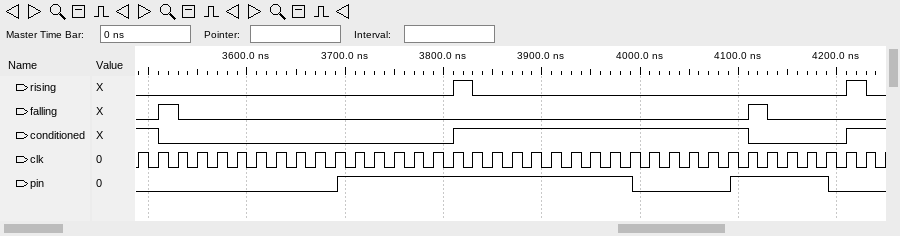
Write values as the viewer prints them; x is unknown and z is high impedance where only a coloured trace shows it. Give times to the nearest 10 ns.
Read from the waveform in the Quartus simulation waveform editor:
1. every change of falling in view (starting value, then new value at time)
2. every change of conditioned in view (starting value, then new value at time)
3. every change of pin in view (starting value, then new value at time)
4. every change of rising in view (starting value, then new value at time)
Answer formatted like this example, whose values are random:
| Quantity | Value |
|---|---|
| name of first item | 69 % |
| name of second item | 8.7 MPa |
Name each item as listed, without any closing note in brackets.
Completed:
| Quantity | Value |
|---|---|
| every change of falling in view | 0, 1 at 3510 ns, 0 at 3530 ns, 1 at 4110 ns, 0 at 4130 ns |
| every change of conditioned in view | 1, 0 at 3510 ns, 1 at 3810 ns, 0 at 4110 ns, 1 at 4210 ns |
| every change of pin in view | 0, 1 at 3690 ns, 0 at 3990 ns, 1 at 4090 ns, 0 at 4190 ns |
| every change of rising in view | 0, 1 at 3810 ns, 0 at 3830 ns, 1 at 4210 ns, 0 at 4230 ns |
